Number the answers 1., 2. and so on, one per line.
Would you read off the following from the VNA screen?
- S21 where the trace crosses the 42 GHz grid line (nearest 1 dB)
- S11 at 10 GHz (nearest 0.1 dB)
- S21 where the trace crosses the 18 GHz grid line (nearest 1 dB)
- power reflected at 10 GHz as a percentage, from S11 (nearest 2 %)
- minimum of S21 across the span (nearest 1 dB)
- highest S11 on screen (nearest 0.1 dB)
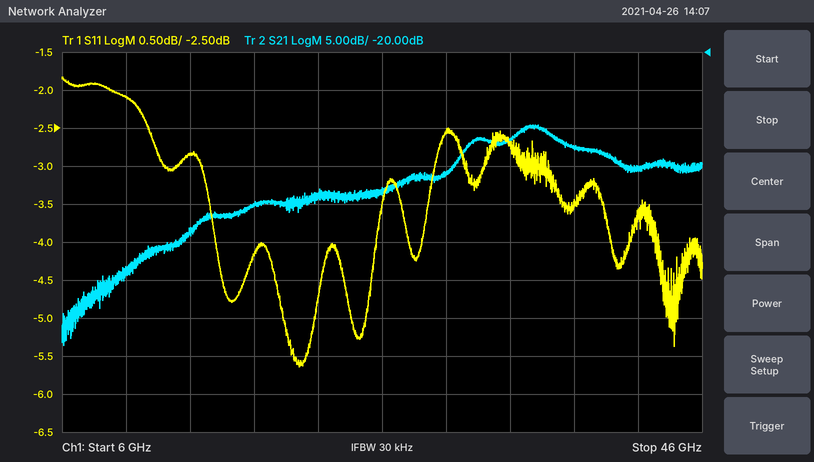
1. -35 dB
2. -2.1 dB
3. -40 dB
4. 62 %
5. -59 dB
6. -1.8 dB
